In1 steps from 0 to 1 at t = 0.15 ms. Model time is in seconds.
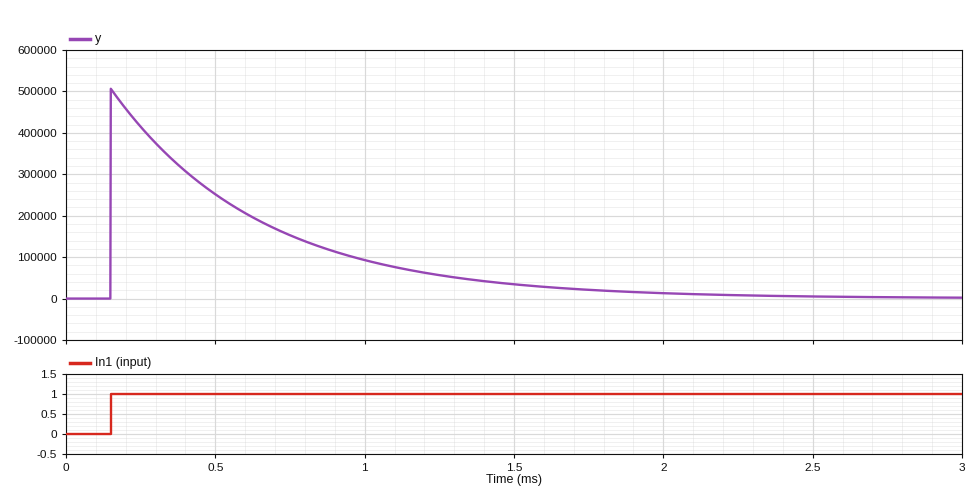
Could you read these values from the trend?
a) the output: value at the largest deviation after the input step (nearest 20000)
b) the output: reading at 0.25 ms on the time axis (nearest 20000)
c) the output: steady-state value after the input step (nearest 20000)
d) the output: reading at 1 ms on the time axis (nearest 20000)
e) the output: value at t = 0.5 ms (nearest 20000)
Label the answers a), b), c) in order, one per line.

a) 500000
b) 420000
c) 0
d) 100000
e) 260000
